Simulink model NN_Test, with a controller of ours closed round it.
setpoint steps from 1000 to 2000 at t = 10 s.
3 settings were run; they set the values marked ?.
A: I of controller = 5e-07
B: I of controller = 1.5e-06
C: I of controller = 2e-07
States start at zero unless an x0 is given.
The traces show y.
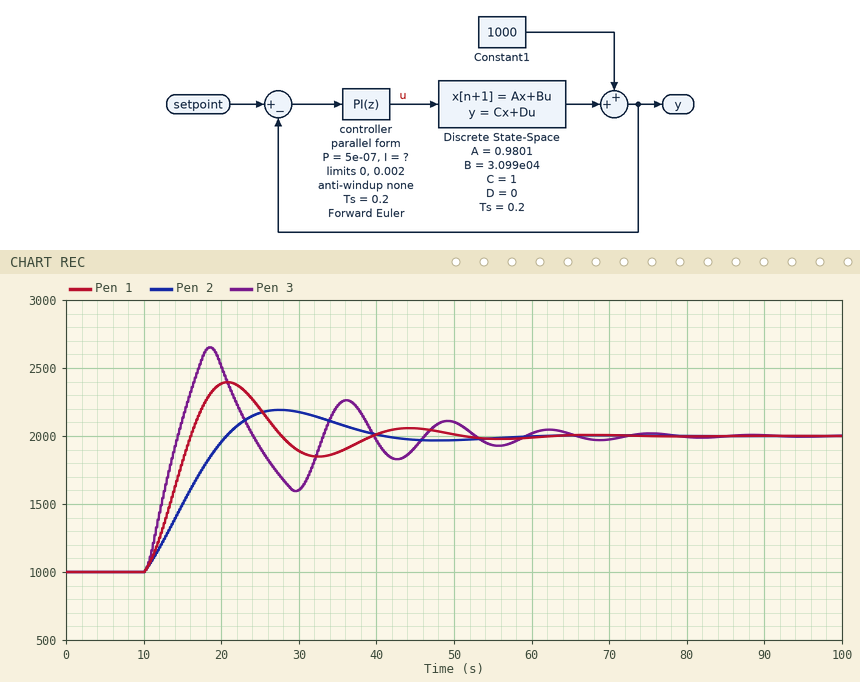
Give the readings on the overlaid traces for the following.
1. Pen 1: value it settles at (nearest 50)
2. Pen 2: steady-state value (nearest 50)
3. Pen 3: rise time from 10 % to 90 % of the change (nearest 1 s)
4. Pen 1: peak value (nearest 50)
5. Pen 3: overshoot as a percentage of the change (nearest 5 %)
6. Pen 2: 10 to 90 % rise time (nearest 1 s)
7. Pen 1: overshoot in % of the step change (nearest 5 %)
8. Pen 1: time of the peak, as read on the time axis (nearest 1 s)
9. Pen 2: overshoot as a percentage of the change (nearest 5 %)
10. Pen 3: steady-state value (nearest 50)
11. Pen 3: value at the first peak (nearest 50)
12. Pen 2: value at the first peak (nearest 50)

2000
2000
3 s
2400
65 %
8 s
40 %
21 s
20 %
2000
2650
2200
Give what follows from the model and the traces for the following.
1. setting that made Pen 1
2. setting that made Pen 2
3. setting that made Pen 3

A
C
B
